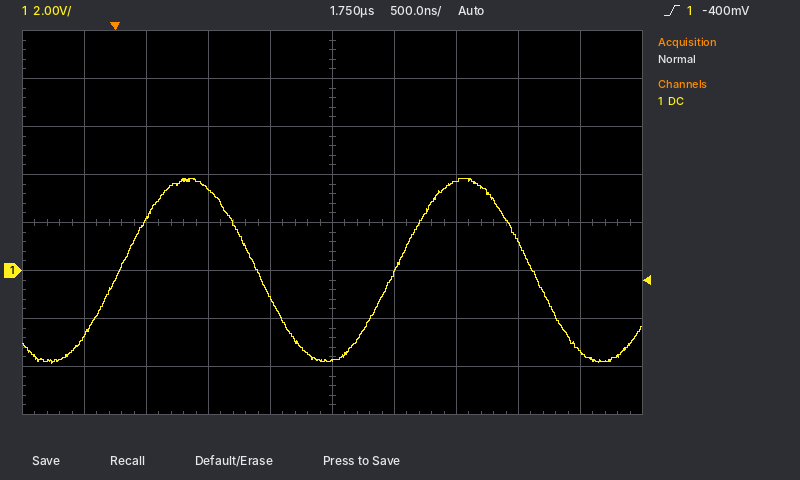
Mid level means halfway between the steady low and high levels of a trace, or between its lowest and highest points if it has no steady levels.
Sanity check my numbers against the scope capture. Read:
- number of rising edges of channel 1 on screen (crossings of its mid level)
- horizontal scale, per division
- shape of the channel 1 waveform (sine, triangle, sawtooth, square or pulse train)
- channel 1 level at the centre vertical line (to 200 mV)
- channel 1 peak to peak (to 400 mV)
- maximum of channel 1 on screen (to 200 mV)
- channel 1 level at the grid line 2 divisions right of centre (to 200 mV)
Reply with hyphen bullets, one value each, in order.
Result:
- 2
- 500 ns
- sine
- -3.8 V
- 7.6 V
- 3.8 V
- 3.8 V
